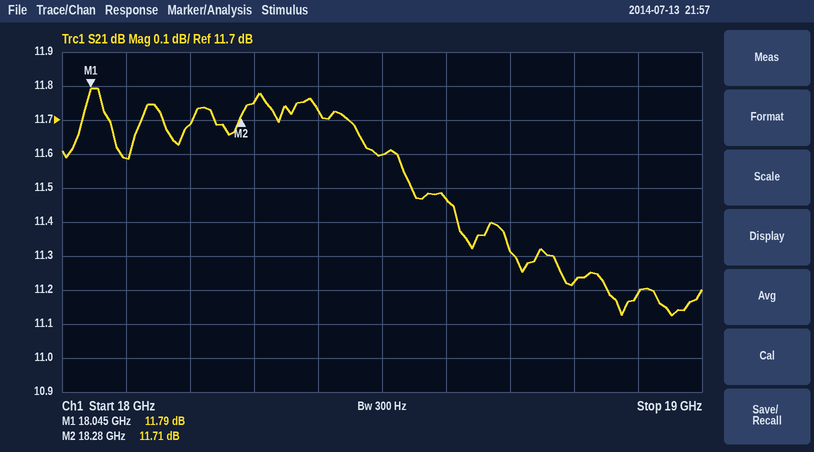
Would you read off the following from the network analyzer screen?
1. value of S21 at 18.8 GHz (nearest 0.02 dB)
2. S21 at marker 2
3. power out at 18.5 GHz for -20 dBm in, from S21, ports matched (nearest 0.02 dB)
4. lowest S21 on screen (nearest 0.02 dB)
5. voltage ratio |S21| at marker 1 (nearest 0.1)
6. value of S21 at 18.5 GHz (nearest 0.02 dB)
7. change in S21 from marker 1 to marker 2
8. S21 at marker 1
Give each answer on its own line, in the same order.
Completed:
11.22 dB
11.71 dB
-8.40 dBm
11.12 dB
3.9
11.60 dB
-0.08 dB
11.79 dB
